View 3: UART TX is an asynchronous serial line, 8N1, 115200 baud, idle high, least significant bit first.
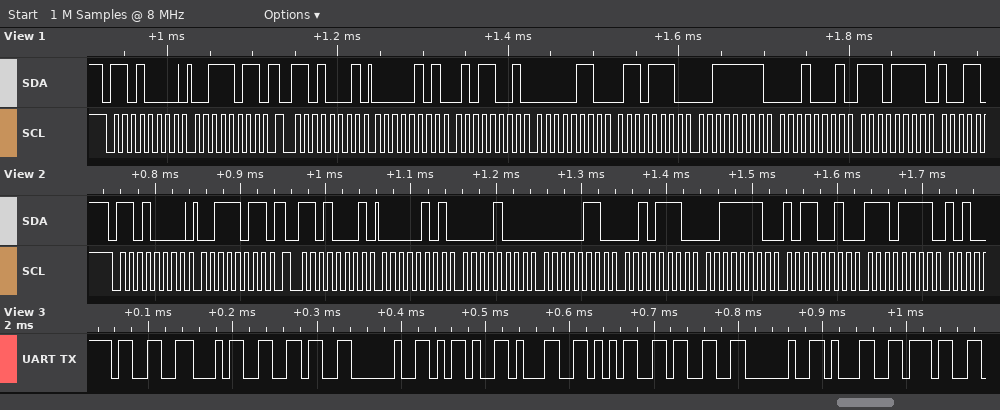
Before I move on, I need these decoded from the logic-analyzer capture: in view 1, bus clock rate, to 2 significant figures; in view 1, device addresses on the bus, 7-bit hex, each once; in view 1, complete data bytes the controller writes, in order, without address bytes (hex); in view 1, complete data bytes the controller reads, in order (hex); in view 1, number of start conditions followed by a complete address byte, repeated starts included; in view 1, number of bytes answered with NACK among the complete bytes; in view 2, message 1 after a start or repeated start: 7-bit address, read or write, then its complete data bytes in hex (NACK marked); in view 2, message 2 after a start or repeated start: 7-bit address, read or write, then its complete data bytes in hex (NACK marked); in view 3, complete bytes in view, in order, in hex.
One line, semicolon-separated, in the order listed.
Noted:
100 kHz; 0x68; 3B; 05 59 06 6E 3F 11 EF; 2; 0; 0x68 write: 3B; 0x68 read: 05 08 06 2E 3E B2 EF; 33 34 36 20 2D 31 35 33 20 31 37
